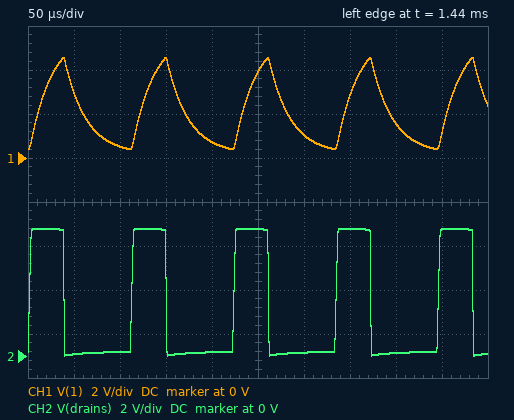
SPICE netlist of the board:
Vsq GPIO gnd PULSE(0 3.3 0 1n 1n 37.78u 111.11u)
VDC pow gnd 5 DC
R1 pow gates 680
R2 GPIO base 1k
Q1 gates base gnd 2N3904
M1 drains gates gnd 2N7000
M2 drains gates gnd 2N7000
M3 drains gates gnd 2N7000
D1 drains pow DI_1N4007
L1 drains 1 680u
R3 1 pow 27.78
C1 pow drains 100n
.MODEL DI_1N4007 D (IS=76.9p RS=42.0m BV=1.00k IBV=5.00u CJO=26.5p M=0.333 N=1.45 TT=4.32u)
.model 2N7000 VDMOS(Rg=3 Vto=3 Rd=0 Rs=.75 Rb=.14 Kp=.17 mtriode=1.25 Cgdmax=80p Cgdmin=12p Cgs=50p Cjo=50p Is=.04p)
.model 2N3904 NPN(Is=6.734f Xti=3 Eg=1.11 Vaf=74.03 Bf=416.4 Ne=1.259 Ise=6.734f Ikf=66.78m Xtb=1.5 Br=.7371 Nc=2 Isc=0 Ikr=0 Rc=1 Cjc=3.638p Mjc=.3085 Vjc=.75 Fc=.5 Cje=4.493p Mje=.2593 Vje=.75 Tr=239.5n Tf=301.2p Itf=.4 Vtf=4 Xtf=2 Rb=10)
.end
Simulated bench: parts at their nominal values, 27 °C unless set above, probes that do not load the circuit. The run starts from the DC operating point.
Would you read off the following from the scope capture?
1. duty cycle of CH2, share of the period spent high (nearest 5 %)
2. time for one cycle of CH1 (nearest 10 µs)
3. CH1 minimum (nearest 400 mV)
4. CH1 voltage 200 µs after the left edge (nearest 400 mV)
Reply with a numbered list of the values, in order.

1. 35 %
2. 110 µs
3. 400 mV
4. 800 mV
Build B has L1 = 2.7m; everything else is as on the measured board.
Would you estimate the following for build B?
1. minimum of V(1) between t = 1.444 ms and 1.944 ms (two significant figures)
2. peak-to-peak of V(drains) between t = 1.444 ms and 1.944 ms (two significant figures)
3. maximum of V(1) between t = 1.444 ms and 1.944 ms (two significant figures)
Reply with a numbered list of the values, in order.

1. 1.4 V
2. 5.7 V
3. 2.8 V
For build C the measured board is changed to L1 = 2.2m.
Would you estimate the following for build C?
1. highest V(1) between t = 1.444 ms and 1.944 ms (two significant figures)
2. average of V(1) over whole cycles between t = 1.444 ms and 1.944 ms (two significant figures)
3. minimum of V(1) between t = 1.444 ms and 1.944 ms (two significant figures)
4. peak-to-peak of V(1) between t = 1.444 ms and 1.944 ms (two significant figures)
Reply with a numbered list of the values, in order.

1. 2.9 V
2. 2.0 V
3. 1.3 V
4. 1.7 V
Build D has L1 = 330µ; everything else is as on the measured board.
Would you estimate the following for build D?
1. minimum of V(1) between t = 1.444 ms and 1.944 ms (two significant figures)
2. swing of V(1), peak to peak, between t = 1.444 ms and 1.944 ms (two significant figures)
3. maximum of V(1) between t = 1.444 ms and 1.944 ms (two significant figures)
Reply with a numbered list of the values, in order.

1. 200 mV
2. 5.1 V
3. 5.3 V
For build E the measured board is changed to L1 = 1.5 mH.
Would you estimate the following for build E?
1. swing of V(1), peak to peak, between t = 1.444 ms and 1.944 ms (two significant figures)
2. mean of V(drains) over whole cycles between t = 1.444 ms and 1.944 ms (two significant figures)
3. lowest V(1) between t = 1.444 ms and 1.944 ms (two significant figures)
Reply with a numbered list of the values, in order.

1. 2.4 V
2. 2.0 V
3. 980 mV
